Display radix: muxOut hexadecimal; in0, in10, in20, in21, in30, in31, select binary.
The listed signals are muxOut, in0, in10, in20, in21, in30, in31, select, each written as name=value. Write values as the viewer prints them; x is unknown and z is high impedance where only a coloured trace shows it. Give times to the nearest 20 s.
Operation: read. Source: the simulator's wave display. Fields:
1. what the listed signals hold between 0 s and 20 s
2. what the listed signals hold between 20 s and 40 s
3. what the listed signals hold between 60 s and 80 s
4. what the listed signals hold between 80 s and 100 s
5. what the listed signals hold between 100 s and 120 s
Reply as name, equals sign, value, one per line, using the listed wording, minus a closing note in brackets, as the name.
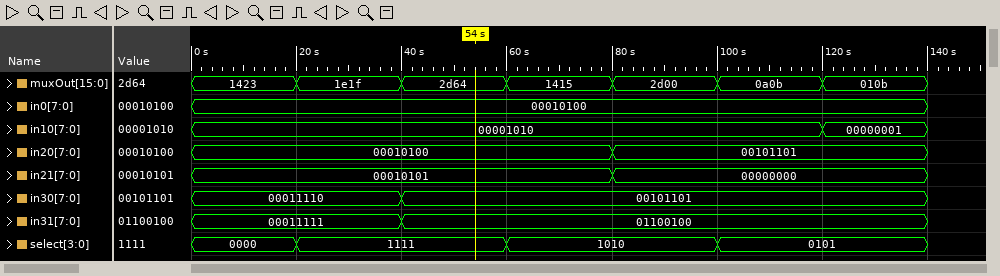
what the listed signals hold between 0 s and 20 s = muxOut=1423, in0=00010100, in10=00001010, in20=00010100, in21=00010101, in30=00011110, in31=00011111, select=0000
what the listed signals hold between 20 s and 40 s = muxOut=1e1f, in0=00010100, in10=00001010, in20=00010100, in21=00010101, in30=00011110, in31=00011111, select=1111
what the listed signals hold between 60 s and 80 s = muxOut=1415, in0=00010100, in10=00001010, in20=00010100, in21=00010101, in30=00101101, in31=01100100, select=1010
what the listed signals hold between 80 s and 100 s = muxOut=2d00, in0=00010100, in10=00001010, in20=00101101, in21=00000000, in30=00101101, in31=01100100, select=1010
what the listed signals hold between 100 s and 120 s = muxOut=0a0b, in0=00010100, in10=00001010, in20=00101101, in21=00000000, in30=00101101, in31=01100100, select=0101
